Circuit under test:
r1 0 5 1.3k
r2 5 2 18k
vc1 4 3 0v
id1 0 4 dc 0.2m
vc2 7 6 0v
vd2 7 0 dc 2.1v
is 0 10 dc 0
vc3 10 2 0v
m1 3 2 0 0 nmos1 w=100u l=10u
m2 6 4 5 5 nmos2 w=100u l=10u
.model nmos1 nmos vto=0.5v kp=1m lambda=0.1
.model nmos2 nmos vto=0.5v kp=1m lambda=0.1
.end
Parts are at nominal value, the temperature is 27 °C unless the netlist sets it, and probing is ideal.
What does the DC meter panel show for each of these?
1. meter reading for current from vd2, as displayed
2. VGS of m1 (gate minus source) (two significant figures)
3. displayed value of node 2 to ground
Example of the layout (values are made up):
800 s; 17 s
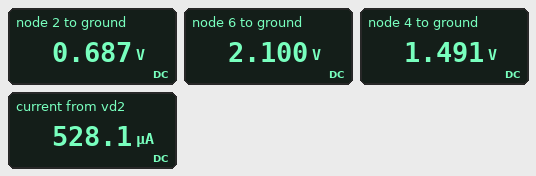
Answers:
528.1 µA; 690 mV; 0.687 V
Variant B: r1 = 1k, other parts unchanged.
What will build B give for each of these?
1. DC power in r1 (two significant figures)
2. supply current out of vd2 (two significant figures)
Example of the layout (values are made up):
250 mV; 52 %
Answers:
470 µW; 690 µA
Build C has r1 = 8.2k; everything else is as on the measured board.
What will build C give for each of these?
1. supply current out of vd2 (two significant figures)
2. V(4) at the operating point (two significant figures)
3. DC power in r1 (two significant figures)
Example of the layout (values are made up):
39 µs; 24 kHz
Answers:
84 µA; 1.3 V; 58 µW
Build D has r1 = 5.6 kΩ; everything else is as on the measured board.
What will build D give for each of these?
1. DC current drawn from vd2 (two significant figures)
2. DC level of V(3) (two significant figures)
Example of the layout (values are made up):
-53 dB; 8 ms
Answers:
120 µA; 1.3 V
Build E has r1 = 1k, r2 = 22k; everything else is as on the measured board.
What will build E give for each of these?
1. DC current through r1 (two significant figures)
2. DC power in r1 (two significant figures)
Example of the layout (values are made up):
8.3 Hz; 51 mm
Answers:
690 µA; 470 µW
